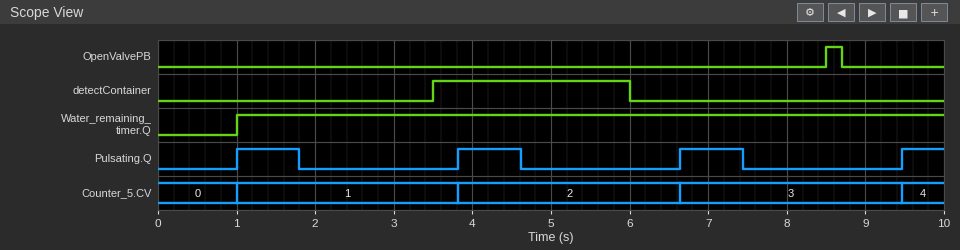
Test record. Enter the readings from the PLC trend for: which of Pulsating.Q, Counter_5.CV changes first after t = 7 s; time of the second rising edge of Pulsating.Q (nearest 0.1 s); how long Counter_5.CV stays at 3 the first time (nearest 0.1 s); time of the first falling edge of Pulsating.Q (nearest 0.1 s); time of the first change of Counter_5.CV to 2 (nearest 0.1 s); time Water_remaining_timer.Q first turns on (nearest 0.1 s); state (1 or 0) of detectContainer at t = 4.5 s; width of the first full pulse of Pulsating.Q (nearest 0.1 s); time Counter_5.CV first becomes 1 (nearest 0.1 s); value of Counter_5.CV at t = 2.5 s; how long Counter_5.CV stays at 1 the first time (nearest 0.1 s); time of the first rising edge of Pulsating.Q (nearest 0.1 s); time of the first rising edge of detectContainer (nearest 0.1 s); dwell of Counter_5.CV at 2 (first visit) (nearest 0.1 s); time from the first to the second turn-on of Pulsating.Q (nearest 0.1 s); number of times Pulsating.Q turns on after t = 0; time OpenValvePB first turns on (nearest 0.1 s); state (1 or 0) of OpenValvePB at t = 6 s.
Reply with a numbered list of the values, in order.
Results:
1. Pulsating.Q
2. 3.8 s
3. 2.8 s
4. 1.8 s
5. 3.8 s
6. 1.0 s
7. 1
8. 0.8 s
9. 1.0 s
10. 1
11. 2.8 s
12. 1.0 s
13. 3.5 s
14. 2.8 s
15. 2.8 s
16. 4
17. 8.5 s
18. 0
